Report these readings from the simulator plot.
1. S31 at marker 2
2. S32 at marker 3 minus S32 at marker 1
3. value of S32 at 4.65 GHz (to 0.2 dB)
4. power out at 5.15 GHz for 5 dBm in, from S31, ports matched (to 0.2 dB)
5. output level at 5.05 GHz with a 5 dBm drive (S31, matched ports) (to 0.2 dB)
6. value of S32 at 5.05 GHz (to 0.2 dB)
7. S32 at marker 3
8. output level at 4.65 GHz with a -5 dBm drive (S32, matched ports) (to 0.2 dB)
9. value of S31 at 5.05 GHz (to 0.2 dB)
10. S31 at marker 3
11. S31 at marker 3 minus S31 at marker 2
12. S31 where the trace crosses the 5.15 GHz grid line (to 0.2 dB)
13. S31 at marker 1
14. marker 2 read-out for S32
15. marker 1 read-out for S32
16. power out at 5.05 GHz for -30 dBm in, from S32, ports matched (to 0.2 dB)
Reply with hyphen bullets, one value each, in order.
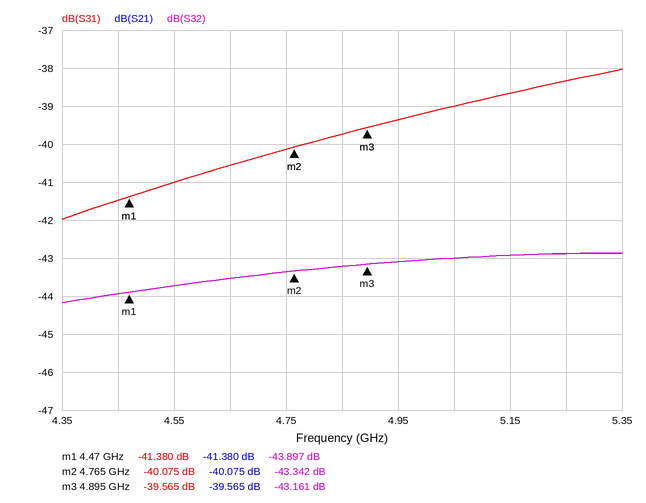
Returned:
- -40.075 dB
- 0.736 dB
- -43.6 dB
- -33.6 dBm
- -34.0 dBm
- -43.0 dB
- -43.161 dB
- -48.6 dBm
- -39.0 dB
- -39.565 dB
- 0.510 dB
- -38.6 dB
- -41.380 dB
- -43.342 dB
- -43.897 dB
- -73.0 dBm
